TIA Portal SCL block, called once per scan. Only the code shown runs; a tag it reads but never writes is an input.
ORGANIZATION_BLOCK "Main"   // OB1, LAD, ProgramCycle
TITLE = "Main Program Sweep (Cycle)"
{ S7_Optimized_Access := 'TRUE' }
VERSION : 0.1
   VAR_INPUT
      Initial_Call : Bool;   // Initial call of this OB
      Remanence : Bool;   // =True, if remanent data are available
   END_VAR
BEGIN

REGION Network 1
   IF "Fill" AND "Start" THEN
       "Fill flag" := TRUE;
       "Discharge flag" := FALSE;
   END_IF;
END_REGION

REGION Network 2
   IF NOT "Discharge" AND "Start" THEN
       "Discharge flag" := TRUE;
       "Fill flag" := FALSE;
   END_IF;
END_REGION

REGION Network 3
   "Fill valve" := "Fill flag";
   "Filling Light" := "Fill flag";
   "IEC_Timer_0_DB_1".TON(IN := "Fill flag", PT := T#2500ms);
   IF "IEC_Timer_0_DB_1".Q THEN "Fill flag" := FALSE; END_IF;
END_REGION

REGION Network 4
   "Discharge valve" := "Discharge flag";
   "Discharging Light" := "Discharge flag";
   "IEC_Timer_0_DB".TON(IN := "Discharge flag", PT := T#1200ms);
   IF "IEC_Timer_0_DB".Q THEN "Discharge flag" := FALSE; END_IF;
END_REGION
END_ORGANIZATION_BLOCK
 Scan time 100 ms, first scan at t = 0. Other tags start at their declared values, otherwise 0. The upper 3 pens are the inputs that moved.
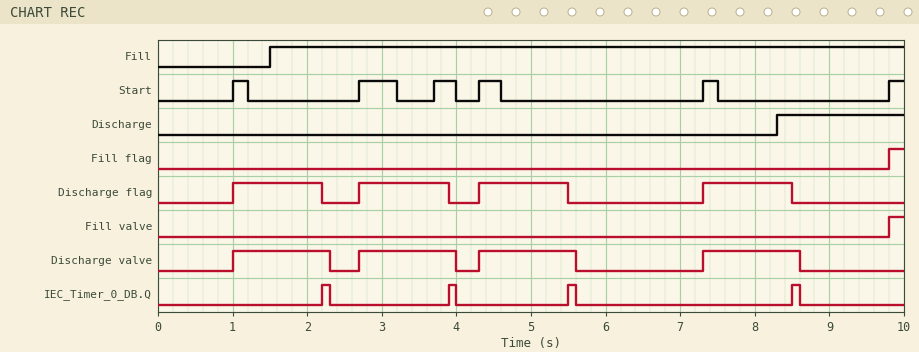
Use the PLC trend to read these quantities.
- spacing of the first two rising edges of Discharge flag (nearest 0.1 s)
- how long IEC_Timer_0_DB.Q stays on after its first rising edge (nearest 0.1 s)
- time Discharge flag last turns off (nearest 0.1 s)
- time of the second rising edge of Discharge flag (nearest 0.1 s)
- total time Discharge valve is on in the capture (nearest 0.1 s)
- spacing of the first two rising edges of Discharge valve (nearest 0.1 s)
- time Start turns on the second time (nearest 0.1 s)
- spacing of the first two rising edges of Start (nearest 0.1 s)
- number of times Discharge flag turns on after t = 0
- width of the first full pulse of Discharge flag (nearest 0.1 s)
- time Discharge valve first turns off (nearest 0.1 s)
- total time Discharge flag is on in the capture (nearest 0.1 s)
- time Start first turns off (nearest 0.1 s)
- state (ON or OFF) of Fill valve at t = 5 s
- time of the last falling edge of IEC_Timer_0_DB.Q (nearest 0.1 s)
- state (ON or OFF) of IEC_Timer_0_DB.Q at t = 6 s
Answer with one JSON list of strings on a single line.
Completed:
["1.7 s", "0.1 s", "8.5 s", "2.7 s", "5.2 s", "1.7 s", "2.7 s", "1.7 s", "4", "1.2 s", "2.3 s", "4.8 s", "1.2 s", "OFF", "8.6 s", "OFF"]
